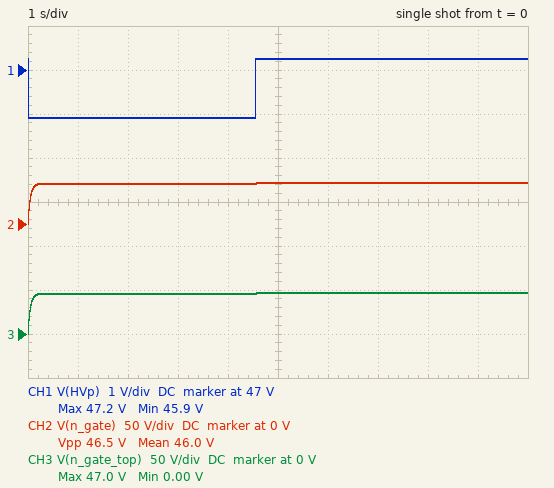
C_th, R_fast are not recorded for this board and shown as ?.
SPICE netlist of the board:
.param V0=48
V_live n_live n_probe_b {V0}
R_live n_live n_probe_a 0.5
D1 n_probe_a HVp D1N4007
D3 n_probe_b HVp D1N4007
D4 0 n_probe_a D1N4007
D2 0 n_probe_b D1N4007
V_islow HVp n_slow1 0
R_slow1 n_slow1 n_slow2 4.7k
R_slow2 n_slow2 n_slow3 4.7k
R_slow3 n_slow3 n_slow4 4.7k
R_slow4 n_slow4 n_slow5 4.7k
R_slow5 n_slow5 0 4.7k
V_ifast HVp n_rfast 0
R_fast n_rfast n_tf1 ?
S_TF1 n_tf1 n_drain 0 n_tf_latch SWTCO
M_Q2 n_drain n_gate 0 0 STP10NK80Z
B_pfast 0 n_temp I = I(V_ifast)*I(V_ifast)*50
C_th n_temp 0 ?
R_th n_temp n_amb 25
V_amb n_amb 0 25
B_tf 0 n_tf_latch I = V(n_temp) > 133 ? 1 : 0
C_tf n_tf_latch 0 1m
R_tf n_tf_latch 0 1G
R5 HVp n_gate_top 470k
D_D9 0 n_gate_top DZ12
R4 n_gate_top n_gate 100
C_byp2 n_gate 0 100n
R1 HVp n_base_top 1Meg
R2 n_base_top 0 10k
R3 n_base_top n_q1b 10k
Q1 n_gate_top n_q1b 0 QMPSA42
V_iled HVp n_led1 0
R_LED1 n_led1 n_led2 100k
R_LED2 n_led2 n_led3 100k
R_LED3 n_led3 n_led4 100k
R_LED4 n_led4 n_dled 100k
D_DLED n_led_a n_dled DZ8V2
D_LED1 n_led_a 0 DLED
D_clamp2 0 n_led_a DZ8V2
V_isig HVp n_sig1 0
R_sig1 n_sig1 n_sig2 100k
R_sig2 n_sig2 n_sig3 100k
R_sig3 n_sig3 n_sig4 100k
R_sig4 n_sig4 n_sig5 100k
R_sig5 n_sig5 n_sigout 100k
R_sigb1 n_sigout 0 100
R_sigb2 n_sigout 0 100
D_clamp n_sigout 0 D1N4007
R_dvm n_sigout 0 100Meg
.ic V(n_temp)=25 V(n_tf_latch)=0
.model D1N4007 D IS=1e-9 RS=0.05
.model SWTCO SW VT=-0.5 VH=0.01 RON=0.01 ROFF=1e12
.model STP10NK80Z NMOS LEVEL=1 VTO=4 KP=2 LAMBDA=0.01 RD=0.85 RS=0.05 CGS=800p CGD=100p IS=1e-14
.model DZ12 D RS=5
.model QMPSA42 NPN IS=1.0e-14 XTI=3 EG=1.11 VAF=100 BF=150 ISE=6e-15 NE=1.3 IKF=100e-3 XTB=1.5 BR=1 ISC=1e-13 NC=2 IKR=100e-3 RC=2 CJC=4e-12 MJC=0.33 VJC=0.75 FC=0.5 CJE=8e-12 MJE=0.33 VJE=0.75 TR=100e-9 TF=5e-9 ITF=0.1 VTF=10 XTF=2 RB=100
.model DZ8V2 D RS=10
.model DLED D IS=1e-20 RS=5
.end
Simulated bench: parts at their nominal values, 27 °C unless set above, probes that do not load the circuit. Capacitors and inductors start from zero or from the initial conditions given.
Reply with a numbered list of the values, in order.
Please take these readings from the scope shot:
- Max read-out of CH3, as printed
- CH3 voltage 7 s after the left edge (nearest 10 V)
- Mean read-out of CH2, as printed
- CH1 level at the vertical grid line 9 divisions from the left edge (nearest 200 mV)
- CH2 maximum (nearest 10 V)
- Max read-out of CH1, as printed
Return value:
1. 47.0 V
2. 50 V
3. 46.0 V
4. 47.2 V
5. 50 V
6. 47.2 V
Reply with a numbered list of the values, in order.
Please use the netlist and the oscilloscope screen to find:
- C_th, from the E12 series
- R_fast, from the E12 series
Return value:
1. 5.6 F
2. 27 Ω
